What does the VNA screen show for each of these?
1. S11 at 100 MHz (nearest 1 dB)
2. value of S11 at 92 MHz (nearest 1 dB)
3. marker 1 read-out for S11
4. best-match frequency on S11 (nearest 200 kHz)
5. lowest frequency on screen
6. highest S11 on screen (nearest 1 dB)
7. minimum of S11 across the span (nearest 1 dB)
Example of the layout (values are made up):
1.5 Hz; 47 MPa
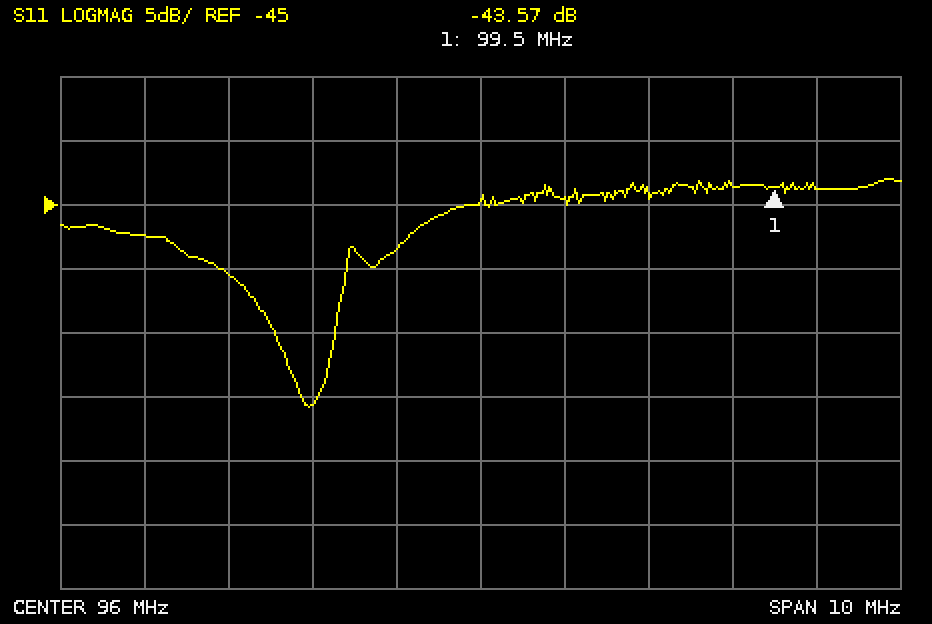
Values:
-44 dB; -47 dB; -43.57 dB; 94.0 MHz; 91 MHz; -43 dB; -61 dB
